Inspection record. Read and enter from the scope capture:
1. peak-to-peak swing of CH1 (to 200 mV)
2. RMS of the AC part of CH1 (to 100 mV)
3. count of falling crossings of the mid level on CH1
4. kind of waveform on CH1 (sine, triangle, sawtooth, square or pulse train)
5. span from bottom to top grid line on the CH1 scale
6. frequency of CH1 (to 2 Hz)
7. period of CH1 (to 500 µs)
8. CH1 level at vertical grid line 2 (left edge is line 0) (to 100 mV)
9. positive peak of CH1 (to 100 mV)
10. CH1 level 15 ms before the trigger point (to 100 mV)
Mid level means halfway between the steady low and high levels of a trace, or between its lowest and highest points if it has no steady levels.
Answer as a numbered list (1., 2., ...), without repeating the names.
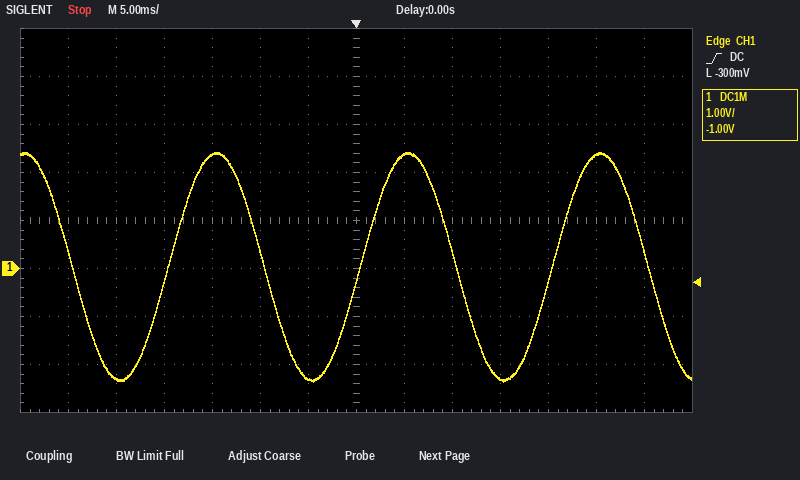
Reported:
1. 4.8 V
2. 1.7 V
3. 4
4. sine
5. 8 V
6. 50 Hz
7. 20.0 ms
8. -2.3 V
9. 2.4 V
10. 2.4 V
